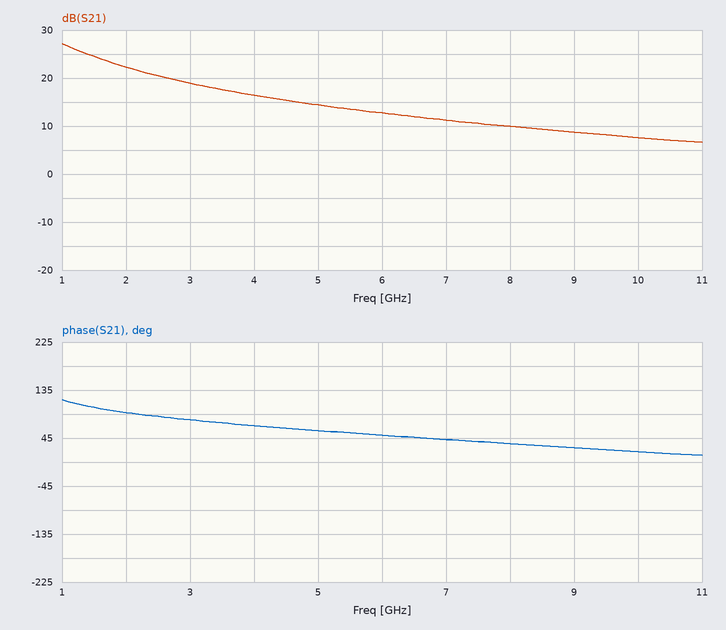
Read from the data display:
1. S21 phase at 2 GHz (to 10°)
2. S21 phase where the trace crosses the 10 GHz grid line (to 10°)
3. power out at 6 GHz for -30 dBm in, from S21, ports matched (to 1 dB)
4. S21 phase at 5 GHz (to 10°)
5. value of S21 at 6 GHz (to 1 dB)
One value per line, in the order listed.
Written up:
90°
20°
-17 dBm
60°
13 dB
